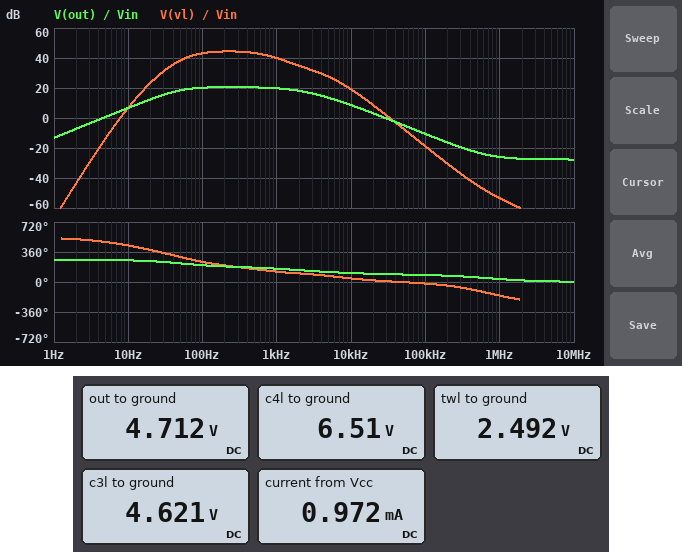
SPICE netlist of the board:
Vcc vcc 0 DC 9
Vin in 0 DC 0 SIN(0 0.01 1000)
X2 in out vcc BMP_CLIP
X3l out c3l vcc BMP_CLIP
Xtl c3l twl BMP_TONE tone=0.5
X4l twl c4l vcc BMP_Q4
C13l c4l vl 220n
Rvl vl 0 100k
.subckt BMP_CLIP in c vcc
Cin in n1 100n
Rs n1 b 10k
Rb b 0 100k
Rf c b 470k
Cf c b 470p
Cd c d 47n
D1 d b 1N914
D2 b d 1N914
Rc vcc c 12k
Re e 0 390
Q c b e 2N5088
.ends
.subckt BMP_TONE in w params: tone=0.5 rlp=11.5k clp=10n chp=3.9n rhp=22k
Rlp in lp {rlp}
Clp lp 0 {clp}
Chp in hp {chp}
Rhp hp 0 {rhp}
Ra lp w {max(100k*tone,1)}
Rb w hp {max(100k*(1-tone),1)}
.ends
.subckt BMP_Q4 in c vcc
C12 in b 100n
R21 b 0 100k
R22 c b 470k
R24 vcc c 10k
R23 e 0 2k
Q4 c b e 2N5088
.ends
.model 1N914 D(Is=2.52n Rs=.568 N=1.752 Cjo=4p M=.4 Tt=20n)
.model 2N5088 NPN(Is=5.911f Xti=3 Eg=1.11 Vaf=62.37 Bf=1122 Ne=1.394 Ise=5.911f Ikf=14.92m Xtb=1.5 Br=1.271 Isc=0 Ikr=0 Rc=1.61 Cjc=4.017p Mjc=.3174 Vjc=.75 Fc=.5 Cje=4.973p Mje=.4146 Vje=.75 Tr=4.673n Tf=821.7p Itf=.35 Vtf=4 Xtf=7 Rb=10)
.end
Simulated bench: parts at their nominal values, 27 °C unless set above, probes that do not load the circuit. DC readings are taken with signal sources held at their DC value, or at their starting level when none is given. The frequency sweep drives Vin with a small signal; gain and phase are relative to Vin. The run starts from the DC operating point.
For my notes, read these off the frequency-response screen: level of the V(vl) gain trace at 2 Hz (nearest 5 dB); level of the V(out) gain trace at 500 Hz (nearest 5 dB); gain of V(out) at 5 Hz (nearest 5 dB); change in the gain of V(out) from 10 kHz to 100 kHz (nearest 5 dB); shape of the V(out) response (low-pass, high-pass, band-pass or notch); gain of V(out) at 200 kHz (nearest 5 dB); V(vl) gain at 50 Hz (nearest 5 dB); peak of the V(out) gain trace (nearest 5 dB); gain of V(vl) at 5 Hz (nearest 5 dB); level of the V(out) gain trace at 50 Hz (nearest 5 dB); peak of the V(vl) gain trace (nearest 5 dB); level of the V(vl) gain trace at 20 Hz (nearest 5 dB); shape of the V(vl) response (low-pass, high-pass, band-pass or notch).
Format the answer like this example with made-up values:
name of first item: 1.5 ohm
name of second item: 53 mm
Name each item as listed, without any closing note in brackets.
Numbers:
level of the V(vl) gain trace at 2 Hz: -45 dB
level of the V(out) gain trace at 500 Hz: 20 dB
gain of V(out) at 5 Hz: 0 dB
change in the gain of V(out) from 10 kHz to 100 kHz: -20 dB
shape of the V(out) response: band-pass
gain of V(out) at 200 kHz: -15 dB
V(vl) gain at 50 Hz: 40 dB
peak of the V(out) gain trace: 20 dB
gain of V(vl) at 5 Hz: -15 dB
level of the V(out) gain trace at 50 Hz: 20 dB
peak of the V(vl) gain trace: 45 dB
level of the V(vl) gain trace at 20 Hz: 25 dB
shape of the V(vl) response: band-pass
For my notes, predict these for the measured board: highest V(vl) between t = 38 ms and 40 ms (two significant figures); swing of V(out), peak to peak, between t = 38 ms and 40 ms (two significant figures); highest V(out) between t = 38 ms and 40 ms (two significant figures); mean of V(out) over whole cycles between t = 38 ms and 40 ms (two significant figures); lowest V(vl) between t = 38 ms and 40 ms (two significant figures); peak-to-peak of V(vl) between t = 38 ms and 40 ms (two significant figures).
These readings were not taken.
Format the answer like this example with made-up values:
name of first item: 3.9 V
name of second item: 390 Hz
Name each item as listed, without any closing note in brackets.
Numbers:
highest V(vl) between t = 38 ms and 40 ms: 380 mV
swing of V(out), peak to peak, between t = 38 ms and 40 ms: 170 mV
highest V(out) between t = 38 ms and 40 ms: 4.8 V
mean of V(out) over whole cycles between t = 38 ms and 40 ms: 4.7 V
lowest V(vl) between t = 38 ms and 40 ms: -380 mV
peak-to-peak of V(vl) between t = 38 ms and 40 ms: 760 mV
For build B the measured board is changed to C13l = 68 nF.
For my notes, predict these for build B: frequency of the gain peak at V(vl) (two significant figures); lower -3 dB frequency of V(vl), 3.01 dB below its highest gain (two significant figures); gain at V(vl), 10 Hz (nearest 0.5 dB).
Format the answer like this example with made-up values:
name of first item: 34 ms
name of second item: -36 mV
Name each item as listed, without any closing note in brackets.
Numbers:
frequency of the gain peak at V(vl): 230 Hz
lower -3 dB frequency of V(vl), 3.01 dB below its highest gain: 74 Hz
gain at V(vl), 10 Hz: 1.0 dB
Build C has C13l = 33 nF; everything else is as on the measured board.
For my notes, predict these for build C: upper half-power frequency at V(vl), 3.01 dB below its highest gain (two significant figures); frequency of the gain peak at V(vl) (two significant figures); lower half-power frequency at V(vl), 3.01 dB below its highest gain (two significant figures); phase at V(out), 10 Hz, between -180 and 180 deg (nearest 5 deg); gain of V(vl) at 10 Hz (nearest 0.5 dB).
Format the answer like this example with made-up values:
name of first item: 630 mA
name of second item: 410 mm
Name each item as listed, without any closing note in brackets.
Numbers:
upper half-power frequency at V(vl), 3.01 dB below its highest gain: 810 Hz
frequency of the gain peak at V(vl): 240 Hz
lower half-power frequency at V(vl), 3.01 dB below its highest gain: 83 Hz
phase at V(out), 10 Hz, between -180 and 180 deg: -100 deg
gain of V(vl) at 10 Hz: -5.0 dB
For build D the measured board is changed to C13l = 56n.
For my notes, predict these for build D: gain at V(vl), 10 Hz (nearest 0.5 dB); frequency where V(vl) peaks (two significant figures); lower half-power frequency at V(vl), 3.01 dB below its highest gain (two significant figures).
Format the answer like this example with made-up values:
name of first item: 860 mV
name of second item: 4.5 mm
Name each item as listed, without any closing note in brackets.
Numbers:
gain at V(vl), 10 Hz: -0.5 dB
frequency where V(vl) peaks: 230 Hz
lower half-power frequency at V(vl), 3.01 dB below its highest gain: 75 Hz
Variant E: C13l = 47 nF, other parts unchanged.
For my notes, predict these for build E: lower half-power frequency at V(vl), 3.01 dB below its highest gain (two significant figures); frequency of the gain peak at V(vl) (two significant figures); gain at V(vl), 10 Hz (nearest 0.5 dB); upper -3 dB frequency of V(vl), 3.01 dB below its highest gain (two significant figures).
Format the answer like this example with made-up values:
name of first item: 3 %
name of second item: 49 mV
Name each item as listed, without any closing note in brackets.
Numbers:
lower half-power frequency at V(vl), 3.01 dB below its highest gain: 77 Hz
frequency of the gain peak at V(vl): 230 Hz
gain at V(vl), 10 Hz: -2.0 dB
upper -3 dB frequency of V(vl), 3.01 dB below its highest gain: 800 Hz
